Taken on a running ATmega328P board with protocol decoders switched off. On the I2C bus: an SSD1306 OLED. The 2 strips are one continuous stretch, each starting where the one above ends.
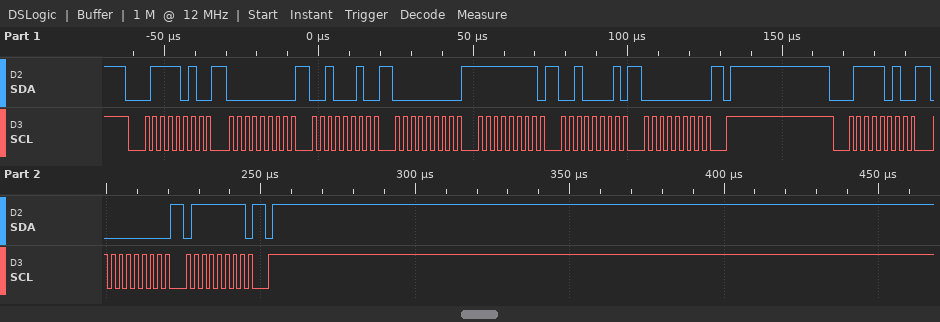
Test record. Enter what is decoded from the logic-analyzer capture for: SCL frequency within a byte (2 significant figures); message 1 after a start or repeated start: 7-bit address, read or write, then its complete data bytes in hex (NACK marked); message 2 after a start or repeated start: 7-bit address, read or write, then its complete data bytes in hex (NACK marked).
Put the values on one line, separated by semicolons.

400 kHz; 0x3D write: 00 22 00 FF 21 00; 0x3D write: 00 7F
